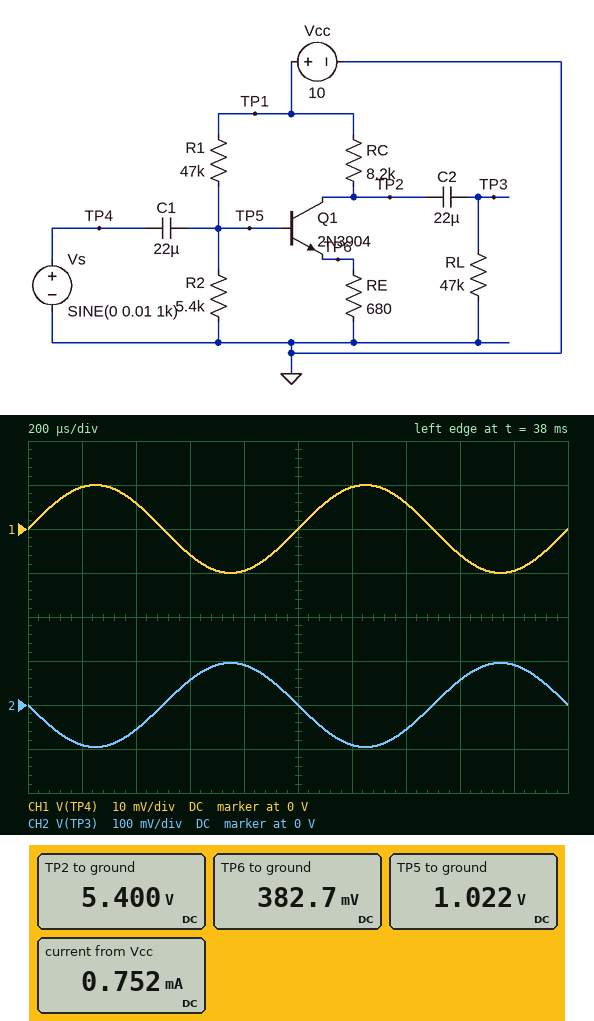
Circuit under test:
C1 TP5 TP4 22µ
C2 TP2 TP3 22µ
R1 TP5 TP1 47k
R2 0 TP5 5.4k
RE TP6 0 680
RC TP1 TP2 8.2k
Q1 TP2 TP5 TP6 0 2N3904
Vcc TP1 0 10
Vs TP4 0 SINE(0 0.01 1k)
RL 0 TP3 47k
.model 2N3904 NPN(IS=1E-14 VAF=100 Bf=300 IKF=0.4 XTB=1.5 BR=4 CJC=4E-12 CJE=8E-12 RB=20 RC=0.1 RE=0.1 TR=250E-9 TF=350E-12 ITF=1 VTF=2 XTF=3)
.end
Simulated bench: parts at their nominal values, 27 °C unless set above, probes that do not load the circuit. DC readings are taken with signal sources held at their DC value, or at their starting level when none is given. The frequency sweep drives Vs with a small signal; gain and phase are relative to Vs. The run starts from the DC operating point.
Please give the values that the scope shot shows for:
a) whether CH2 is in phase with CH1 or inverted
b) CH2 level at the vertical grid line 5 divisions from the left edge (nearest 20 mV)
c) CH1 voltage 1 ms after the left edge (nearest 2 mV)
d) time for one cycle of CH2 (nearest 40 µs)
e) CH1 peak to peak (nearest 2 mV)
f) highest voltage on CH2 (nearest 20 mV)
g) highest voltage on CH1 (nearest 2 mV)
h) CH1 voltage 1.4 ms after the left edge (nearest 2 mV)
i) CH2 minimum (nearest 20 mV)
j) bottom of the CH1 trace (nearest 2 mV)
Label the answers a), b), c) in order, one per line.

a) inverted
b) 0 V
c) 0 V
d) 1.00 ms
e) 20 mV
f) 100 mV
g) 10 mV
h) 6 mV
i) -100 mV
j) -10 mV
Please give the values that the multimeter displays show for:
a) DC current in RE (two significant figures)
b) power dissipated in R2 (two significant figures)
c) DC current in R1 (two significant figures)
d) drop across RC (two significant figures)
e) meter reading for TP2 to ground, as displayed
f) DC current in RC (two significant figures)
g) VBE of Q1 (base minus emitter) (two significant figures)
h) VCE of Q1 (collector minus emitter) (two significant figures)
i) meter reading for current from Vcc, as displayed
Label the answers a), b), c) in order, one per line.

a) 560 µA
b) 190 µW
c) 190 µA
d) 4.6 V
e) 5.400 V
f) 560 µA
g) 640 mV
h) 5.0 V
i) 0.752 mA
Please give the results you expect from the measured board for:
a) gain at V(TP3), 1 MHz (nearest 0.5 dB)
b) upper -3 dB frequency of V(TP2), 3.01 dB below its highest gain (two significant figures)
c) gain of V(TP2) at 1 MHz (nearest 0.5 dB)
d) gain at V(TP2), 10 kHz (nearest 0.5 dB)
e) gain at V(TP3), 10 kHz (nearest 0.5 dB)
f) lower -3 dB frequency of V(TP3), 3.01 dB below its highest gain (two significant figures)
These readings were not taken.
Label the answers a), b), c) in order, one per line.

a) 19.5 dB
b) 11 MHz
c) 19.5 dB
d) 19.5 dB
e) 19.5 dB
f) 1.5 Hz
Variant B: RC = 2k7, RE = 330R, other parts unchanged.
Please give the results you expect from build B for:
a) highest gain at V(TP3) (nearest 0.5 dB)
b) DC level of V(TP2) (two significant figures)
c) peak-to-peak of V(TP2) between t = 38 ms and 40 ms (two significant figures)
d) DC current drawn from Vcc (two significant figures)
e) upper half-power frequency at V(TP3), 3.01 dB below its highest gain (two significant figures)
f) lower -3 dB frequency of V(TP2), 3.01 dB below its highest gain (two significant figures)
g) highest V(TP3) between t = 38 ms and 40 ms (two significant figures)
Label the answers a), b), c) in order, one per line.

a) 17.0 dB
b) 7.1 V
c) 140 mV
d) 1.3 mA
e) 31 MHz
f) 1.6 Hz
g) 72 mV
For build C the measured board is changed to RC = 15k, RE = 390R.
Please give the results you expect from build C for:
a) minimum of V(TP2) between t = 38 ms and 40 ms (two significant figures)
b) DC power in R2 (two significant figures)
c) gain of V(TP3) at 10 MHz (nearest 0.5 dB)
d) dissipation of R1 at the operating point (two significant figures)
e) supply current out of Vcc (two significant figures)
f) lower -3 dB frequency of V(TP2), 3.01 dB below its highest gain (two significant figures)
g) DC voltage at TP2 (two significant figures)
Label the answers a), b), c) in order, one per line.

a) 310 mV
b) 150 µW
c) -0.5 dB
d) 1.8 mW
e) 840 µA
f) 14 Hz
g) 320 mV
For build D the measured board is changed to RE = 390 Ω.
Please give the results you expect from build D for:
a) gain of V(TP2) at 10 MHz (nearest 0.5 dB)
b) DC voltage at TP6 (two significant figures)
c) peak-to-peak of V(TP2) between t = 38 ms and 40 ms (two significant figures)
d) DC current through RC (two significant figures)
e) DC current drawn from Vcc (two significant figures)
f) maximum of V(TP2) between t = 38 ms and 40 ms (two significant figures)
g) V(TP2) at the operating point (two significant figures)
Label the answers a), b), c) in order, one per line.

a) 20.0 dB
b) 360 mV
c) 330 mV
d) 930 µA
e) 1.1 mA
f) 2.6 V
g) 2.4 V
